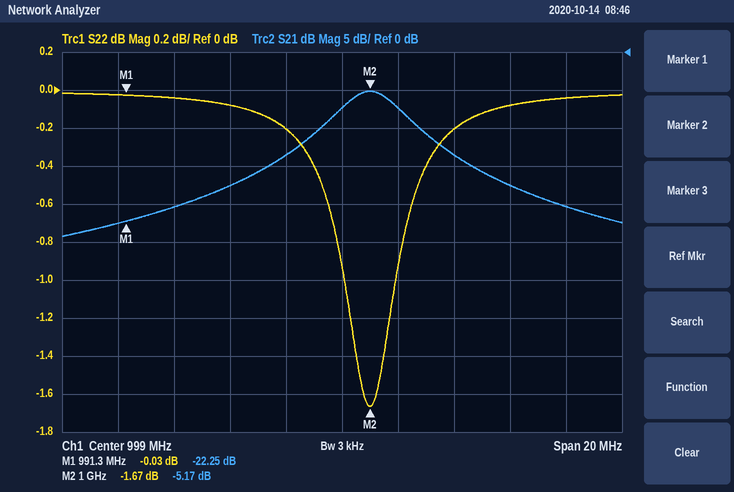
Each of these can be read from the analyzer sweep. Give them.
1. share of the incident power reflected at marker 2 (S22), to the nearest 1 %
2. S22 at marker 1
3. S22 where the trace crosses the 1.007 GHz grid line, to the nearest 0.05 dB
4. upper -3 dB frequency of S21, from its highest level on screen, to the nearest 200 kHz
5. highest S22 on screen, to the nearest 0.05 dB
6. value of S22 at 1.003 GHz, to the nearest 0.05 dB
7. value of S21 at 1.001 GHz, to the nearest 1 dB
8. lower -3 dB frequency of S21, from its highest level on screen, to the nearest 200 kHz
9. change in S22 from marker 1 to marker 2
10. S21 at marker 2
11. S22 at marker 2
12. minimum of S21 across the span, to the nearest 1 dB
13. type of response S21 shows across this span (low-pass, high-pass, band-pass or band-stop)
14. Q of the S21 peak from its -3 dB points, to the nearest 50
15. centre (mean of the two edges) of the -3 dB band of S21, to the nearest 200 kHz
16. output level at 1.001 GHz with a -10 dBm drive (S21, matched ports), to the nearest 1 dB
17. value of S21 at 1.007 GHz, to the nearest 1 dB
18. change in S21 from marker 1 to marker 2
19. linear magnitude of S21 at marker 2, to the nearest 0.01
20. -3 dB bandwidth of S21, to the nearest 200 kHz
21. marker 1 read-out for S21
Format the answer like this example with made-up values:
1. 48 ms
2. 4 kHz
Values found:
1. 68 %
2. -0.03 dB
3. -0.05 dB
4. 1.0012 GHz
5. 0.00 dB
6. -0.20 dB
7. -7 dB
8. 998.8 MHz
9. -1.64 dB
10. -5.17 dB
11. -1.67 dB
12. -24 dB
13. band-pass
14. 400
15. 1.0000 GHz
16. -17 dBm
17. -20 dB
18. 17.08 dB
19. 0.55
20. 2.4 MHz
21. -22.25 dB
